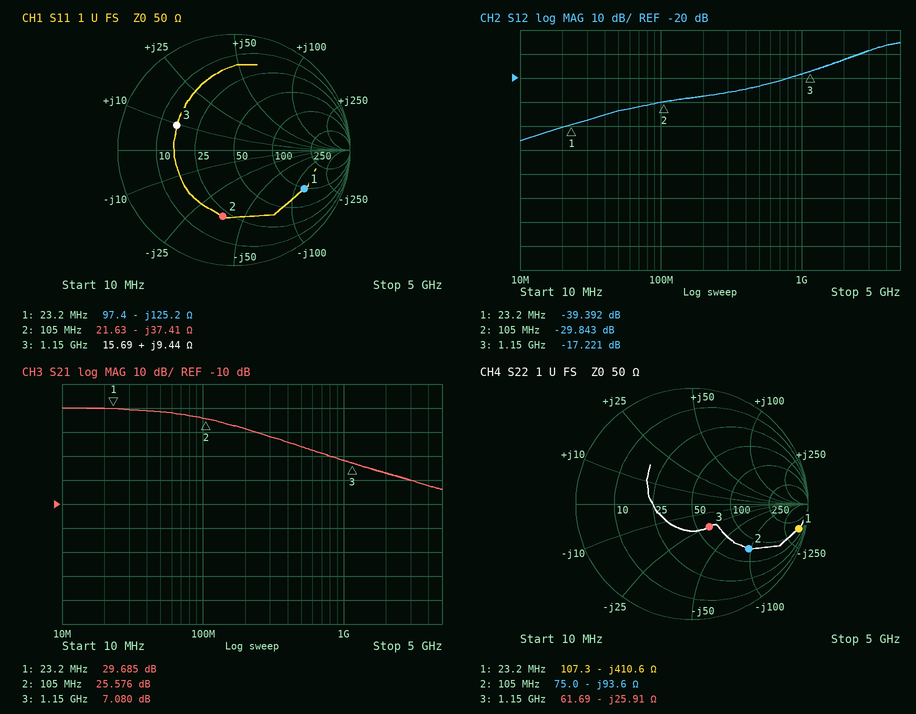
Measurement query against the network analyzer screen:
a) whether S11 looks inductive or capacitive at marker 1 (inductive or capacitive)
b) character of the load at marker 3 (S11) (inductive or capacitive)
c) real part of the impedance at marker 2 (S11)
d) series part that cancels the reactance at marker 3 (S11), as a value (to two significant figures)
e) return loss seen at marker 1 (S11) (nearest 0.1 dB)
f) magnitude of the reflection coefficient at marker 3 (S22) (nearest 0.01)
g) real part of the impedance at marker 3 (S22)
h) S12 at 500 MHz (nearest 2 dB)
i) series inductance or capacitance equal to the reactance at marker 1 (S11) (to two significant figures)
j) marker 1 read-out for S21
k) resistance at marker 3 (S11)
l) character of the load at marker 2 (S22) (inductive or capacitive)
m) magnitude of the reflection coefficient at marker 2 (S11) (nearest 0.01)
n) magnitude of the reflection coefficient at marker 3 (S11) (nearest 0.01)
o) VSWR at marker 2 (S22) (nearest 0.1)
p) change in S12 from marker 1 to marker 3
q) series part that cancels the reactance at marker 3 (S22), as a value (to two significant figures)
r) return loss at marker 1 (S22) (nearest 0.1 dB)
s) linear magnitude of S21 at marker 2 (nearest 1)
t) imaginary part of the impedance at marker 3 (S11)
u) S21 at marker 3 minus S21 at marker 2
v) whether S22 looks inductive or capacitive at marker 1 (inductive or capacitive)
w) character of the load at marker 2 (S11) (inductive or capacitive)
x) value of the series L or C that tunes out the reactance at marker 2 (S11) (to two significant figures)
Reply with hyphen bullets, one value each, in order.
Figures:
- capacitive
- inductive
- 21.63 Ω
- 15 pF
- 3.2 dB
- 0.25
- 61.69 Ω
- -24 dB
- 55 pF
- 29.685 dB
- 15.69 Ω
- capacitive
- 0.58
- 0.54
- 4.3
- 22.171 dB
- 3.6 nH
- 0.5 dB
- 19
- +9.44 Ω
- -18.496 dB
- capacitive
- capacitive
- 57 nH
